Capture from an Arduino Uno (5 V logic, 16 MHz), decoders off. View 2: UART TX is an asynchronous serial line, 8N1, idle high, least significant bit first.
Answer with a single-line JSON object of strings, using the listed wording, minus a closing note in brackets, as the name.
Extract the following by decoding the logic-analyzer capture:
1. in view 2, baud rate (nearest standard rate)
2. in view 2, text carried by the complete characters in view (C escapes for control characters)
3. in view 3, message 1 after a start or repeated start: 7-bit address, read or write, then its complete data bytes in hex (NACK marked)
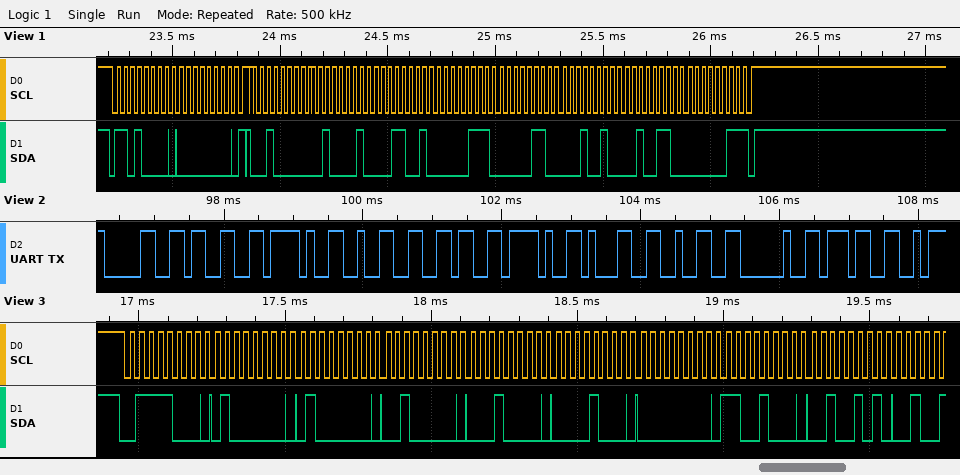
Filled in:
{"in view 2, baud rate": "9600 baud", "in view 2, text carried by the complete characters in view": "\"03/26/12 7\"", "in view 3, message 1 after a start or repeated start: 7-bit address, read or write, then its complete data bytes in hex": "0x3C write: 40 40 20 10 08 00 C8 25"}
